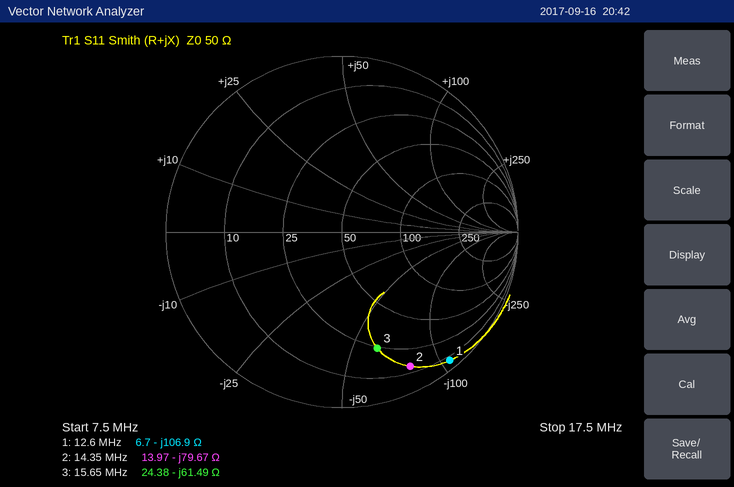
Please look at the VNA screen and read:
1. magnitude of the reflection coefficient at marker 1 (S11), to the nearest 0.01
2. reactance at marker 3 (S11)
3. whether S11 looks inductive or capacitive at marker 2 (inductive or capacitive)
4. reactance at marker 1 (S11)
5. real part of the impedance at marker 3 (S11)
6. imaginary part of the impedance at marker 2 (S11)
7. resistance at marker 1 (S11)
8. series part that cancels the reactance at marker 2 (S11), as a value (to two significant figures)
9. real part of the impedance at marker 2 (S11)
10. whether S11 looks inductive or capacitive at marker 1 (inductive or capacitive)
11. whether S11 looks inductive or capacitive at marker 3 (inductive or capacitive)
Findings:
0.95
-61.49 Ω
capacitive
-106.9 Ω
24.38 Ω
-79.67 Ω
6.7 Ω
880 nH
13.97 Ω
capacitive
capacitive
